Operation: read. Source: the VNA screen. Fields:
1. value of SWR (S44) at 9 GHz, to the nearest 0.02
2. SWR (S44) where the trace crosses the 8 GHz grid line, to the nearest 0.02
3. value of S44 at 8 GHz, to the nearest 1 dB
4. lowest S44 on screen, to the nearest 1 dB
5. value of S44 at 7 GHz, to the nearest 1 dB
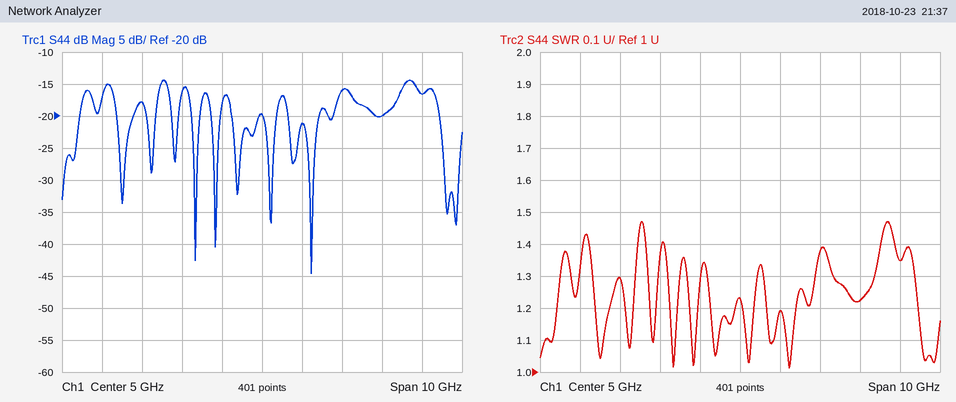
1.34
1.22
-20 dB
-45 dB
-16 dB
